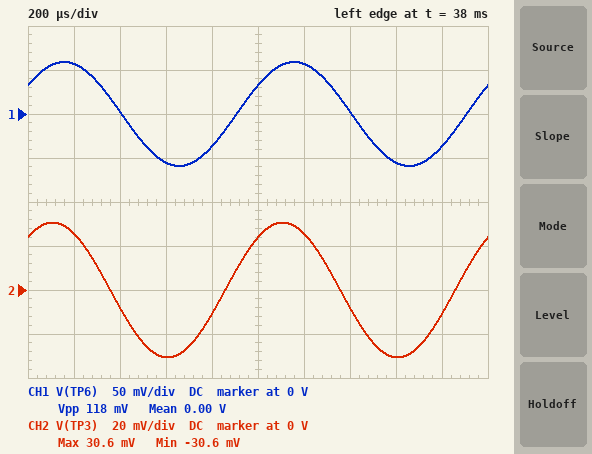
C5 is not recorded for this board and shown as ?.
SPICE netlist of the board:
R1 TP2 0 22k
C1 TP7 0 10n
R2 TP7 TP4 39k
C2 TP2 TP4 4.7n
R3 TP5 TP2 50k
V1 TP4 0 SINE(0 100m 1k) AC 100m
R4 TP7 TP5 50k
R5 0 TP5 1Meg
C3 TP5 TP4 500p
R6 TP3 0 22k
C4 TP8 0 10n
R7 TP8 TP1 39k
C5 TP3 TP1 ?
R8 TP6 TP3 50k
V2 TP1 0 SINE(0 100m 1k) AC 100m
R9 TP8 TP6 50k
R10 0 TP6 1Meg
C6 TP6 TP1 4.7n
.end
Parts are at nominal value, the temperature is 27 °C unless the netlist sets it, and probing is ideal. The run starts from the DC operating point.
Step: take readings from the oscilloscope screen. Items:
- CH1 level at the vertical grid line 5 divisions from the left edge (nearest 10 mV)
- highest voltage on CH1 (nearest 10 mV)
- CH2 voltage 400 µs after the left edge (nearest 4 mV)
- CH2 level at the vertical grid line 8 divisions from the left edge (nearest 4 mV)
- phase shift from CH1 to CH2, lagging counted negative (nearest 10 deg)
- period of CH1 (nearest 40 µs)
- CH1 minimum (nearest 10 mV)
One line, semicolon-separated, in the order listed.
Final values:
30 mV; 60 mV; -8 mV; -32 mV; 20 deg; 1.00 ms; -60 mV
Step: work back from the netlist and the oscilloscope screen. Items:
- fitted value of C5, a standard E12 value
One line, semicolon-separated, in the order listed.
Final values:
1.8 nF
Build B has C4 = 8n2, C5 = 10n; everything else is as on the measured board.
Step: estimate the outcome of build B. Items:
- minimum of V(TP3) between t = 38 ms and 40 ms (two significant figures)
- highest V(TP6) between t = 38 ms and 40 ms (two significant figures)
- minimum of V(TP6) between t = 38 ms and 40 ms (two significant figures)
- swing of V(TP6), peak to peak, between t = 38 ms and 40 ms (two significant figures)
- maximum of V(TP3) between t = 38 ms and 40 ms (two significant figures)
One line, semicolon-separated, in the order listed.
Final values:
-76 mV; 74 mV; -74 mV; 150 mV; 76 mV
